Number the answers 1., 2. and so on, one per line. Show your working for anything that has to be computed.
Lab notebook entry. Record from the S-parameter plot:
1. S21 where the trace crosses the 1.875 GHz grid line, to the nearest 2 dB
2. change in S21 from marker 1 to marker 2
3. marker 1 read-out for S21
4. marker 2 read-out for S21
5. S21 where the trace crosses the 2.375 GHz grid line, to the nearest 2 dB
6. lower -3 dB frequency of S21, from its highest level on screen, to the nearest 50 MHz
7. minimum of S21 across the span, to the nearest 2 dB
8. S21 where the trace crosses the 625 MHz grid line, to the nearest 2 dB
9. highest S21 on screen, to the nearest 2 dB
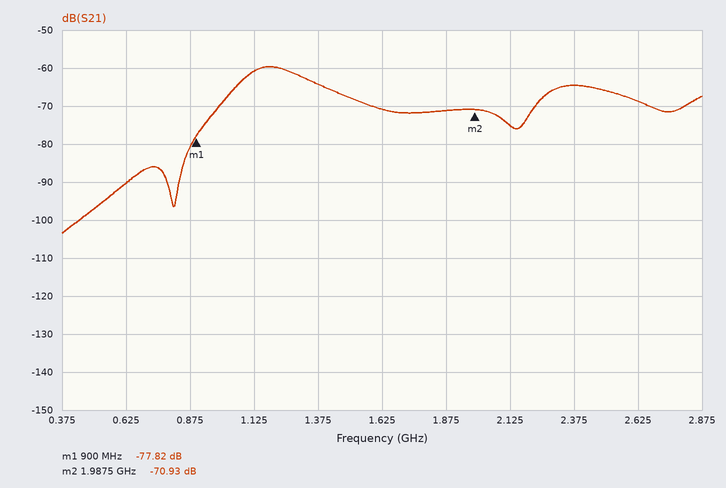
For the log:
1. -72 dB
2. -70.93 − (-77.82) = 6.89 dB
3. -77.82 dB
4. -70.93 dB
5. -64 dB
6. 1.10 GHz
7. -104 dB
8. -90 dB
9. -60 dB
